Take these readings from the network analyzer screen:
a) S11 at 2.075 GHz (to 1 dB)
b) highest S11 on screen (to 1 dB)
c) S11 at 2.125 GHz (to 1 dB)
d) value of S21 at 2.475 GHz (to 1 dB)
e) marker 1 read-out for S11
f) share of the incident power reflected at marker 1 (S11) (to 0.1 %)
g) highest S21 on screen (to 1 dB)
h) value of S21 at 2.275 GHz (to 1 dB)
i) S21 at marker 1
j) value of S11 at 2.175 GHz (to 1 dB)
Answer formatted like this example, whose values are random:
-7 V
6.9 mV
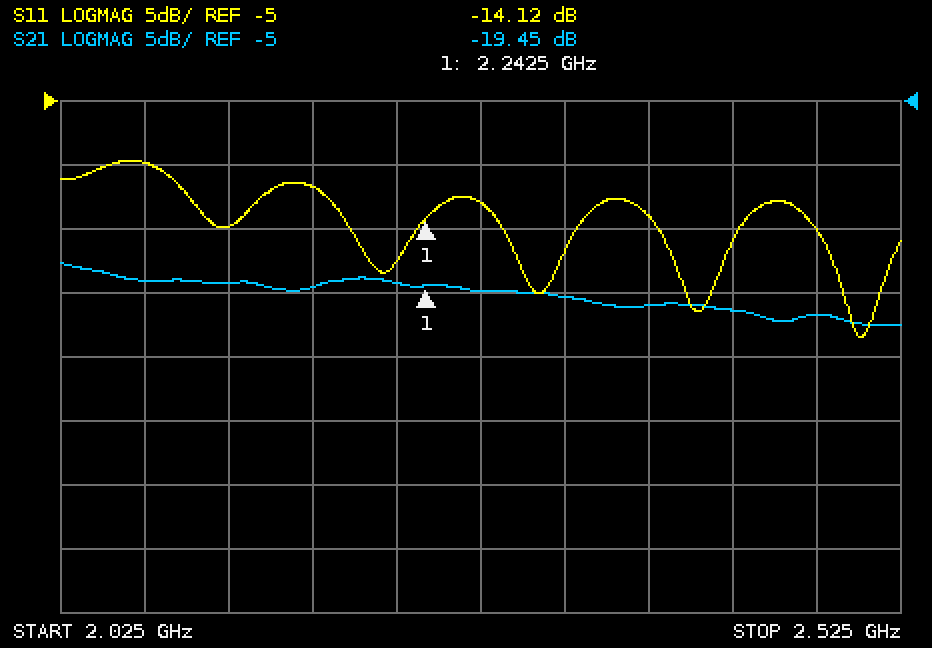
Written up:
-10 dB
-10 dB
-15 dB
-22 dB
-14.12 dB
3.9 %
-18 dB
-20 dB
-19.45 dB
-12 dB
